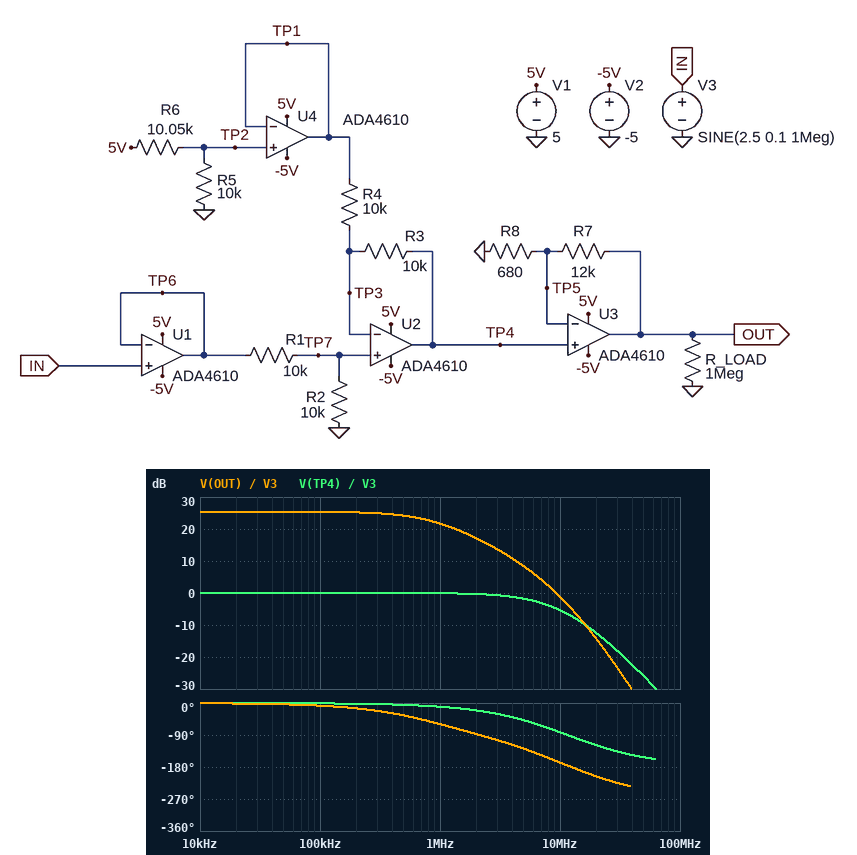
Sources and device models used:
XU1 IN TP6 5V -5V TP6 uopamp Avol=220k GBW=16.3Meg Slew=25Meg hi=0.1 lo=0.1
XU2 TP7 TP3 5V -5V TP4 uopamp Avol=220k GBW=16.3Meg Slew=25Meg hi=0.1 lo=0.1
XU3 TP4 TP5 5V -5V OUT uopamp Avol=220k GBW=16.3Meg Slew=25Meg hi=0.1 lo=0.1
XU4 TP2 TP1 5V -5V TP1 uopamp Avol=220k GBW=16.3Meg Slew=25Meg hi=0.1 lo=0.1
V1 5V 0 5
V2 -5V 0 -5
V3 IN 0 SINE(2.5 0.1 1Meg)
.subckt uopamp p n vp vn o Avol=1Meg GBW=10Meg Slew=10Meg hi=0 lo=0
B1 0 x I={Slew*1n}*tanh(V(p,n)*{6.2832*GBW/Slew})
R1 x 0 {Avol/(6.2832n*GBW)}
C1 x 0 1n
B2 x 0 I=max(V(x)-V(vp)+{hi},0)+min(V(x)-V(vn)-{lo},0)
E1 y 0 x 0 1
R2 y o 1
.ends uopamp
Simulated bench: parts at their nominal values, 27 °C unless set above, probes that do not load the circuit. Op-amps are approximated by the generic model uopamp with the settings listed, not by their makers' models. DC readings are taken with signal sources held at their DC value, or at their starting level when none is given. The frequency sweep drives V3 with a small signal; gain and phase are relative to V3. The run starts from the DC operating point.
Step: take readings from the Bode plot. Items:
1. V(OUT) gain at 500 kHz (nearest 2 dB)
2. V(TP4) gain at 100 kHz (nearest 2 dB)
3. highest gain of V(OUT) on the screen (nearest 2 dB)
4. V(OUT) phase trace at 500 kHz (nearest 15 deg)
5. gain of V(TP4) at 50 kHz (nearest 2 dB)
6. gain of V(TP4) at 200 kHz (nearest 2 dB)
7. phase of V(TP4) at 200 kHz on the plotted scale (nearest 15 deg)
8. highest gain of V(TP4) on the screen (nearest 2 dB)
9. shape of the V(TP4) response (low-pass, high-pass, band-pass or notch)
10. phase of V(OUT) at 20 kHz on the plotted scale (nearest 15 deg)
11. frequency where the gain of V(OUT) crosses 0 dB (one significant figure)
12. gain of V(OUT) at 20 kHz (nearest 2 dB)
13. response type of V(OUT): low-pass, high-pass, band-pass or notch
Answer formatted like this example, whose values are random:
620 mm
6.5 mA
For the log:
24 dB
0 dB
26 dB
-30 deg
0 dB
0 dB
0 deg
0 dB
low-pass
0 deg
9 MHz
26 dB
low-pass
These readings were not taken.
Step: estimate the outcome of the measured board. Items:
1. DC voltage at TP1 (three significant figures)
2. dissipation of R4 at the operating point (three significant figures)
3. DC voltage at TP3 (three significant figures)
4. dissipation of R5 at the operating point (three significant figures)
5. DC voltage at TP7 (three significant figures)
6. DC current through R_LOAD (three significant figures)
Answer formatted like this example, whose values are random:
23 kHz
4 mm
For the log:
2.49 V
155 µW
1.25 V
622 µW
1.25 V
116 nA
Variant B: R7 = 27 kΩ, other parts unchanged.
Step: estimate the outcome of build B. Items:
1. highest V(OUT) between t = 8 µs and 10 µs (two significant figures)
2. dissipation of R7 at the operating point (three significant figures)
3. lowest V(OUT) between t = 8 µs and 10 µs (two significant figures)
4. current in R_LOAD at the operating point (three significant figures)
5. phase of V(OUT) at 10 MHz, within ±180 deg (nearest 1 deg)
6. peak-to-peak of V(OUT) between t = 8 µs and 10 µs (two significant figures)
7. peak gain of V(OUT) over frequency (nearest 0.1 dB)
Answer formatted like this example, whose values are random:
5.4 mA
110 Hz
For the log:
1.7 V
2.27 µW
-1.2 V
254 nA
-170 deg
2.9 V
32.2 dB
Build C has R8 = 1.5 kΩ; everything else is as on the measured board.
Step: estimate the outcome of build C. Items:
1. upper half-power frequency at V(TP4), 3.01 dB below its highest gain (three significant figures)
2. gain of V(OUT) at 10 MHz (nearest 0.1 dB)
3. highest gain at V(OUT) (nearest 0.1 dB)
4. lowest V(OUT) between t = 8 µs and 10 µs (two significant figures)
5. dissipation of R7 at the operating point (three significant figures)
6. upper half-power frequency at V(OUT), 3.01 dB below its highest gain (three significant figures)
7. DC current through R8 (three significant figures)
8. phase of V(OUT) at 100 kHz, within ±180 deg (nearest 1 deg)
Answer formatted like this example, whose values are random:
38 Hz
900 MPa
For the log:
6.83 MHz
-1.3 dB
19.1 dB
-720 mV
207 nW
1.71 MHz
4.16 µA
-4 deg
